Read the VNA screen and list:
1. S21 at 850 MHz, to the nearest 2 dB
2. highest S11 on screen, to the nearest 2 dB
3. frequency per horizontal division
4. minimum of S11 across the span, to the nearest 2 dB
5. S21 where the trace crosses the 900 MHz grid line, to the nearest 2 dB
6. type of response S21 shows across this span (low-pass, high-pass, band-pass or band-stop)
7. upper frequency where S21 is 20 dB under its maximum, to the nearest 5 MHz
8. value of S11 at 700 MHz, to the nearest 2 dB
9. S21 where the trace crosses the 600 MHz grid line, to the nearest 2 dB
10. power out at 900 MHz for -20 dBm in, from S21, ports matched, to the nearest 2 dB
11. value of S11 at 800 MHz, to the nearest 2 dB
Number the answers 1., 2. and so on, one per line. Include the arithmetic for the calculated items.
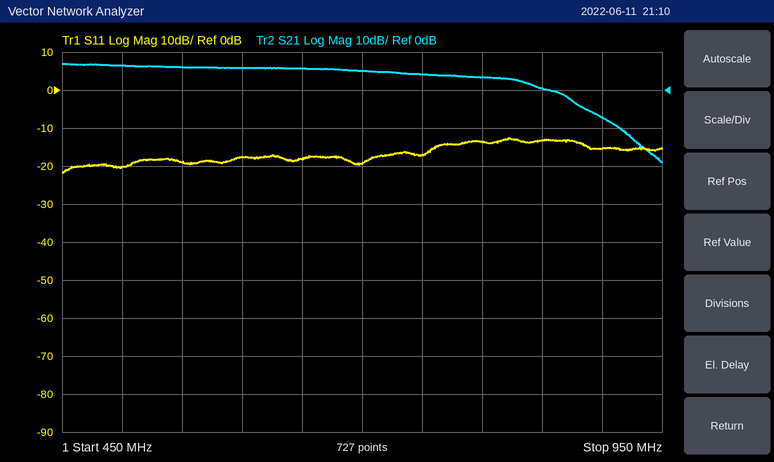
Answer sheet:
1. 0 dB
2. -12 dB
3. 50 MHz
4. -22 dB
5. -8 dB
6. low-pass
7. 925 MHz
8. -20 dB
9. 6 dB
10. -20 dBm + (-8 dB) = -28 dBm
11. -14 dB
